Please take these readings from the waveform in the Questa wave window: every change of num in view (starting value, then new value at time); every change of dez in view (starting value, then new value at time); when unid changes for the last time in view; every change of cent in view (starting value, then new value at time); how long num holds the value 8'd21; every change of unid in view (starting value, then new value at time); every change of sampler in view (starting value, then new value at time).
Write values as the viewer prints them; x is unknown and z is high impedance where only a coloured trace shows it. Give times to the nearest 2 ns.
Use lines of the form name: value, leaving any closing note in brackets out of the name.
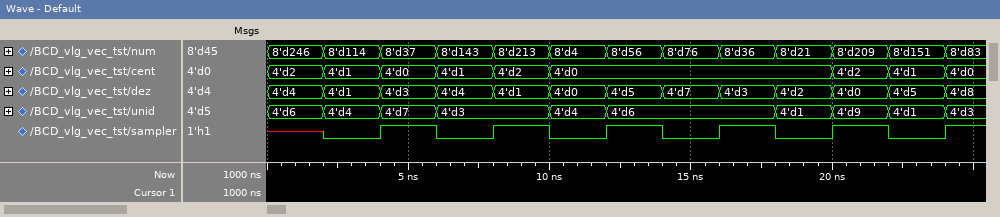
every change of num in view: 8'd246, 8'd114 at 2 ns, 8'd37 at 4 ns, 8'd143 at 6 ns, 8'd213 at 8 ns, 8'd4 at 10 ns, 8'd56 at 12 ns, 8'd76 at 14 ns, 8'd36 at 16 ns, 8'd21 at 18 ns, 8'd209 at 20 ns, 8'd151 at 22 ns, 8'd83 at 24 ns
every change of dez in view: 4'd4, 4'd1 at 2 ns, 4'd3 at 4 ns, 4'd4 at 6 ns, 4'd1 at 8 ns, 4'd0 at 10 ns, 4'd5 at 12 ns, 4'd7 at 14 ns, 4'd3 at 16 ns, 4'd2 at 18 ns, 4'd0 at 20 ns, 4'd5 at 22 ns, 4'd8 at 24 ns
when unid changes for the last time in view: 24 ns
every change of cent in view: 4'd2, 4'd1 at 2 ns, 4'd0 at 4 ns, 4'd1 at 6 ns, 4'd2 at 8 ns, 4'd0 at 10 ns, 4'd2 at 20 ns, 4'd1 at 22 ns, 4'd0 at 24 ns
how long num holds the value 8'd21: 2 ns
every change of unid in view: 4'd6, 4'd4 at 2 ns, 4'd7 at 4 ns, 4'd3 at 6 ns, 4'd4 at 10 ns, 4'd6 at 12 ns, 4'd1 at 18 ns, 4'd9 at 20 ns, 4'd1 at 22 ns, 4'd3 at 24 ns
every change of sampler in view: x, 0 at 2 ns, 1 at 4 ns, 0 at 6 ns, 1 at 8 ns, 0 at 10 ns, 1 at 12 ns, 0 at 14 ns, 1 at 16 ns, 0 at 18 ns, 1 at 20 ns, 0 at 22 ns, 1 at 24 ns
